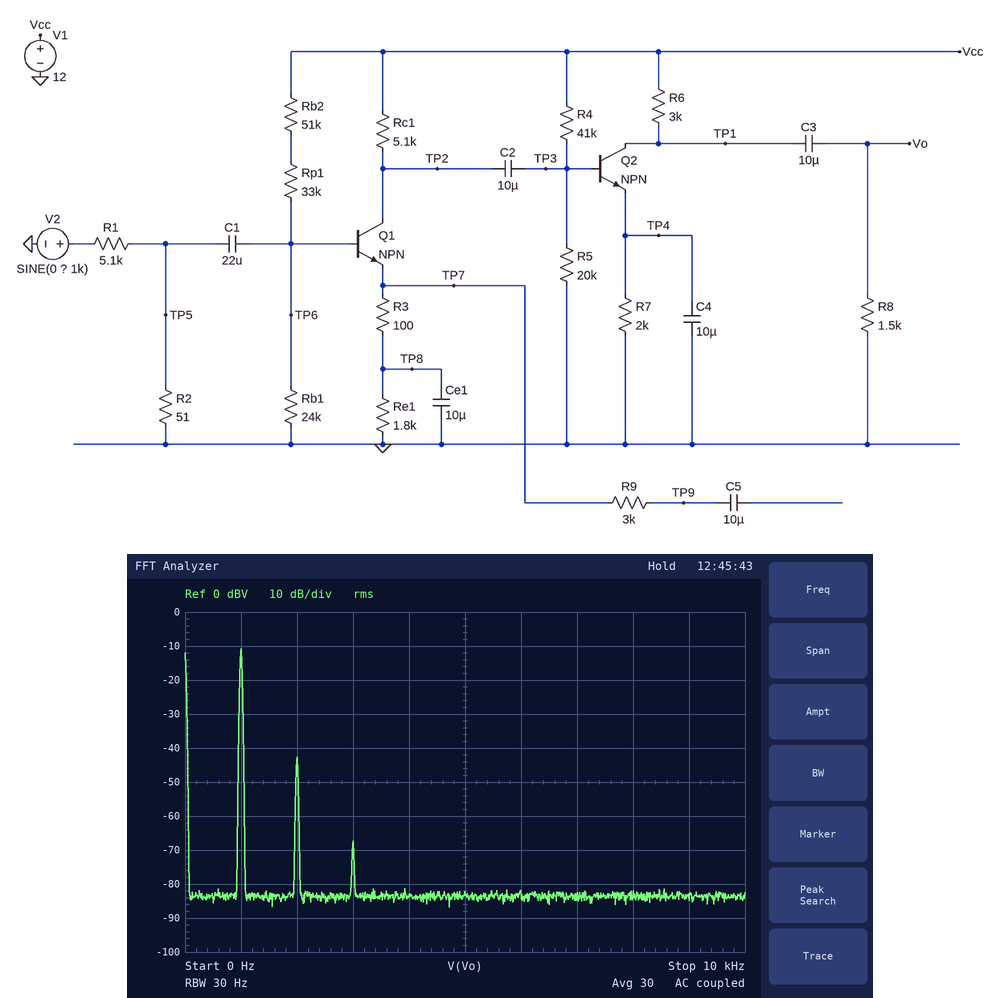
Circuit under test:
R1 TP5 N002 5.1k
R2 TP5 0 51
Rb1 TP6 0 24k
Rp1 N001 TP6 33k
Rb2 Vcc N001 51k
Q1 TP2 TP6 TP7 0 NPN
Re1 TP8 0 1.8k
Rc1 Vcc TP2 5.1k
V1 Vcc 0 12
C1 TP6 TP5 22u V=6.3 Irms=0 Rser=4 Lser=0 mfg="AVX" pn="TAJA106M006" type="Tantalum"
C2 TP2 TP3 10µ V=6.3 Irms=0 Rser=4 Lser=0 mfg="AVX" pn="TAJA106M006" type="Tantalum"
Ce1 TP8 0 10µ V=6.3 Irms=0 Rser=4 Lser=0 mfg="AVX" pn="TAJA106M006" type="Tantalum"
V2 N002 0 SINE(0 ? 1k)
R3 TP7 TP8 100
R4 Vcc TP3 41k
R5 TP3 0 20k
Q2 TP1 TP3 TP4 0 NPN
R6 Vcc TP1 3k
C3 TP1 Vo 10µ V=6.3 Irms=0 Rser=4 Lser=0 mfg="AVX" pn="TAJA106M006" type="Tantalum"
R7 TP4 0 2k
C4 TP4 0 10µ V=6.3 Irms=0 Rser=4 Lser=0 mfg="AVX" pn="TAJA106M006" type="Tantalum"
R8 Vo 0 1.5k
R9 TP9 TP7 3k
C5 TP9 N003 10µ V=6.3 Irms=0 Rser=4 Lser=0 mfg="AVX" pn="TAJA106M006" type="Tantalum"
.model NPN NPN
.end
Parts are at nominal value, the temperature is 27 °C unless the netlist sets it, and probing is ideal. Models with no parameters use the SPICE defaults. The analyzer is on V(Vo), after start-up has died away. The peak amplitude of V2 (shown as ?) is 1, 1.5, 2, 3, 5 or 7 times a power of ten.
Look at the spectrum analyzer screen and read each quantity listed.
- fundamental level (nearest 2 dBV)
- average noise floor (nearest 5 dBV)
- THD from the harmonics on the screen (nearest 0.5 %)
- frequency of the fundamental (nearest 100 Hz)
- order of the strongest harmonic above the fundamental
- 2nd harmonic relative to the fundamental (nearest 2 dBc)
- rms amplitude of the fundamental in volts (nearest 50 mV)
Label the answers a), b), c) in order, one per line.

a) -10 dBV
b) -85 dBV
c) 2.5 %
d) 1.0 kHz
e) 2
f) -32 dBc
g) 300 mV
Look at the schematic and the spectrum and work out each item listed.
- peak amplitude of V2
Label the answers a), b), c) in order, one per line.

a) 100 mV
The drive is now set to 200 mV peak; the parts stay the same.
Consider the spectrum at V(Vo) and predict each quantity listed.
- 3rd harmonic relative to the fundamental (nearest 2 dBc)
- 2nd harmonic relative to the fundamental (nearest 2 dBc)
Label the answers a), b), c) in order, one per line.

a) -44 dBc
b) -26 dBc
